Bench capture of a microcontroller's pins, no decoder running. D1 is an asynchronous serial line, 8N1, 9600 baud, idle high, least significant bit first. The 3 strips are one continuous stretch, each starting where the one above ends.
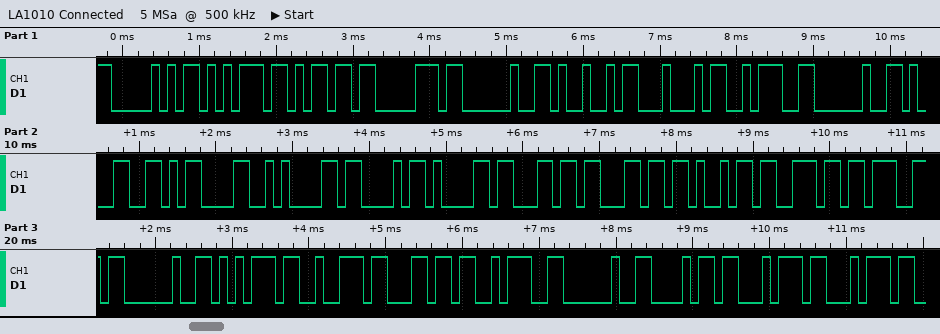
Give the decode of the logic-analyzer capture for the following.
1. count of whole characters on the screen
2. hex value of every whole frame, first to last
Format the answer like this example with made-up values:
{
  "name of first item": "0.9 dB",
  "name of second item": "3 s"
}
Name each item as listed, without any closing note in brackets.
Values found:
{
  "count of whole characters on the screen": "28",
  "hex value of every whole frame, first to last": "50 75 6D 70 20 49 44 3A 20 31 0D 0A 43 61 6C 6C 69 6E 67 20 75 72 6C 3A 20 68 74 74"
}
